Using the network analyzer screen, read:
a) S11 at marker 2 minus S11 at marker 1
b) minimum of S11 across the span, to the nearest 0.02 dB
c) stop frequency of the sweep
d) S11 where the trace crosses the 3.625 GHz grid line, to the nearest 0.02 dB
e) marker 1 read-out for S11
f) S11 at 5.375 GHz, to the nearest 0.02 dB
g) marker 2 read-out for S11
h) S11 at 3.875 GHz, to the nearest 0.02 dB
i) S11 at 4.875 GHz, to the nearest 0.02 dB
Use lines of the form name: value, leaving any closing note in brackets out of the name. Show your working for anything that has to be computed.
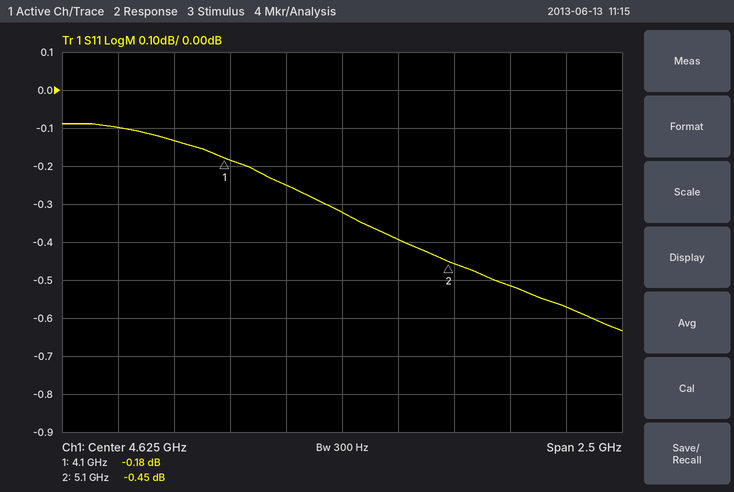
S11 at marker 2 minus S11 at marker 1: -0.45 − (-0.18) = -0.27 dB
minimum of S11 across the span, to the nearest 0.02 dB: -0.64 dB
stop frequency of the sweep: 5.875 GHz
S11 where the trace crosses the 3.625 GHz grid line, to the nearest 0.02 dB: -0.10 dB
marker 1 read-out for S11: -0.18 dB
S11 at 5.375 GHz, to the nearest 0.02 dB: -0.52 dB
marker 2 read-out for S11: -0.45 dB
S11 at 3.875 GHz, to the nearest 0.02 dB: -0.14 dB
S11 at 4.875 GHz, to the nearest 0.02 dB: -0.40 dB
